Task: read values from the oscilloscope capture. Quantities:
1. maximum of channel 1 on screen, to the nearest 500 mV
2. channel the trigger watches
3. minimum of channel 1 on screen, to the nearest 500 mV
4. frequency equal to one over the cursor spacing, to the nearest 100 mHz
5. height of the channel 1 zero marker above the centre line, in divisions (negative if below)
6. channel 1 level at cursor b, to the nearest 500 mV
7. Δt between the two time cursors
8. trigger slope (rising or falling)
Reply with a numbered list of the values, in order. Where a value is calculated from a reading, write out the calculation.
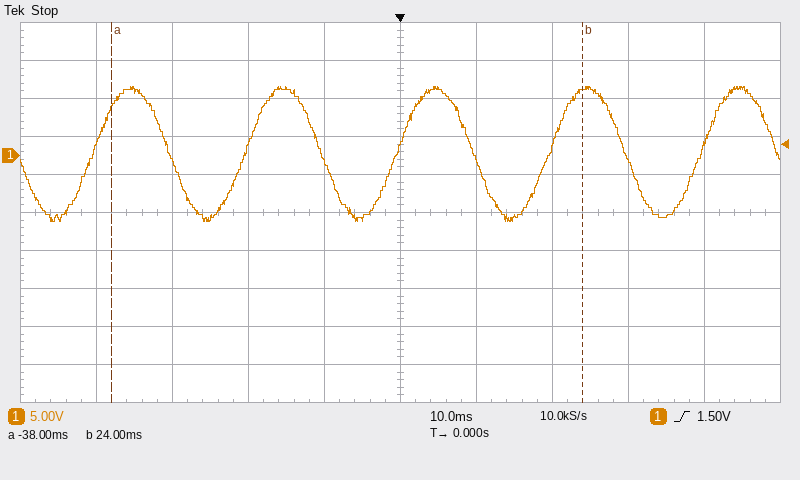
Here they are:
1. 9.0 V
2. channel 1
3. -8.5 V
4. 1 / 62 ms ≈ 16.1 Hz
5. +1.5 div
6. 8.5 V
7. 24 ms − (-38 ms) = 62 ms
8. rising
